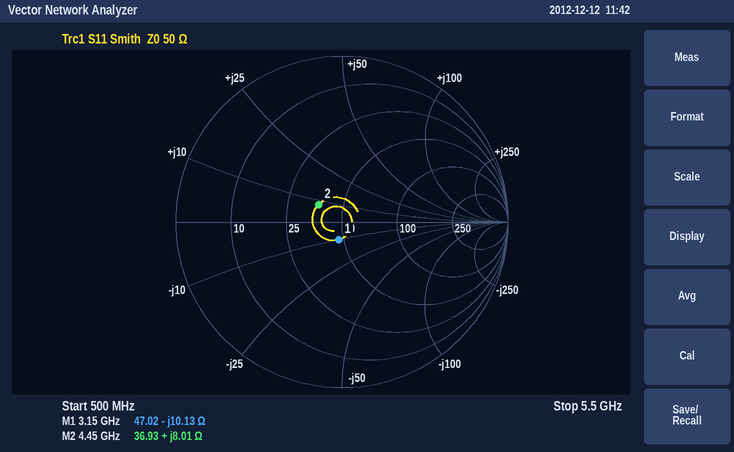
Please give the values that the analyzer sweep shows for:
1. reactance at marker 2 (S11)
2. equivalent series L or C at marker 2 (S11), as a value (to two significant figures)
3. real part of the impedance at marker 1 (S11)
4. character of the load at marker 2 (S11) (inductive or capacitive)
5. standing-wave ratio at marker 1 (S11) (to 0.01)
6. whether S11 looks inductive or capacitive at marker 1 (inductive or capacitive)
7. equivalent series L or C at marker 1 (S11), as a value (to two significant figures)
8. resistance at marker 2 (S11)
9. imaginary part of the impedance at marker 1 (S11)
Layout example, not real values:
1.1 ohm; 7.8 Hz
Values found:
+8.01 Ω; 290 pH; 47.02 Ω; inductive; 1.24; capacitive; 5.0 pF; 36.93 Ω; -10.13 Ω
